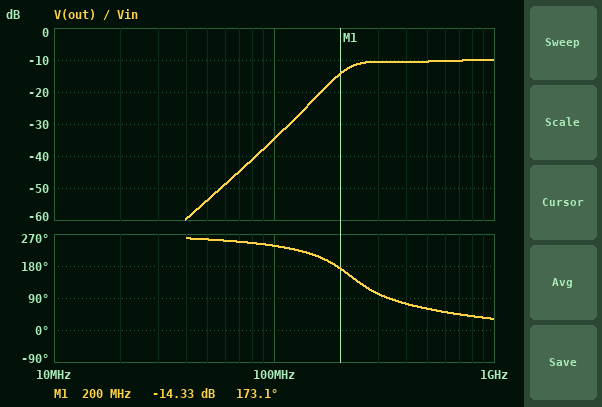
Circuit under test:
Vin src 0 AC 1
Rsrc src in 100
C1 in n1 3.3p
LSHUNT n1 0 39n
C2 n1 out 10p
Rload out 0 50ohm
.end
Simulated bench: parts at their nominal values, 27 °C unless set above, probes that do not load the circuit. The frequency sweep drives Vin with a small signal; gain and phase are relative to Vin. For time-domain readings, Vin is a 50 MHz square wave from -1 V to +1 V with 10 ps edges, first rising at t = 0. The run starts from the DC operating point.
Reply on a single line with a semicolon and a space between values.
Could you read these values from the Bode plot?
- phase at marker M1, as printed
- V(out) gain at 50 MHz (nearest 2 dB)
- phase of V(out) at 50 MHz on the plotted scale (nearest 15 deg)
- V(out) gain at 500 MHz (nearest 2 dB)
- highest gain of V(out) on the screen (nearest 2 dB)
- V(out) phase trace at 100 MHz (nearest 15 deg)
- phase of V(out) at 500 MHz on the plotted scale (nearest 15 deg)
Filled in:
173.1 deg; -54 dB; 255 deg; -10 dB; -10 dB; 240 deg; 60 deg
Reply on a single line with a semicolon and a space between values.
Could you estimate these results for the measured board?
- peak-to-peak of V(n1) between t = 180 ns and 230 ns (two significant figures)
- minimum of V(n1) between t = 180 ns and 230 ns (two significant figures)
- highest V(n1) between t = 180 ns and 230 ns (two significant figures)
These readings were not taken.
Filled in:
1.3 V; -660 mV; 660 mV
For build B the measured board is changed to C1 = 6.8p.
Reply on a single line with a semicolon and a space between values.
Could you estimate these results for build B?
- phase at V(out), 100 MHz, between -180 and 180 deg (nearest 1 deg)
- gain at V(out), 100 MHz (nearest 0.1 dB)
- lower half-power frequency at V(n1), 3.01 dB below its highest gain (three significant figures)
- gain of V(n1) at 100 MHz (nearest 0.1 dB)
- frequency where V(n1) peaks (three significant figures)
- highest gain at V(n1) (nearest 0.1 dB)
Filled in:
-137 deg; -28.6 dB; 164 MHz; -18.1 dB; 224 MHz; -4.8 dB
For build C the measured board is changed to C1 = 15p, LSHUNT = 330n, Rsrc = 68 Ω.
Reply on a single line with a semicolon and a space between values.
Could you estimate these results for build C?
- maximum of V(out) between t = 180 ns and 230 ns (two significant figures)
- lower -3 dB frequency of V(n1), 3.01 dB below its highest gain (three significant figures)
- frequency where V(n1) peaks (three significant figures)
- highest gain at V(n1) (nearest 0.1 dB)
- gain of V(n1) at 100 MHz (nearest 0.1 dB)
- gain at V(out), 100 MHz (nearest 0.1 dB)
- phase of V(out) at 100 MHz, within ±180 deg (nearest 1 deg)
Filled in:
640 mV; 49.9 MHz; 56.7 MHz; 6.6 dB; -1.8 dB; -12.2 dB; 79 deg
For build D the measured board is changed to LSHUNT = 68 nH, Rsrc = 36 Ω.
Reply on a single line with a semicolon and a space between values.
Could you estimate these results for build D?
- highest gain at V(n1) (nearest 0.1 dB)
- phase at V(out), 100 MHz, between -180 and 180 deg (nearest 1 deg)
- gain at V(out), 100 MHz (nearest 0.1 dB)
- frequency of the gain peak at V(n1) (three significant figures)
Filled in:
-3.3 dB; -119 deg; -28.1 dB; 180 MHz
